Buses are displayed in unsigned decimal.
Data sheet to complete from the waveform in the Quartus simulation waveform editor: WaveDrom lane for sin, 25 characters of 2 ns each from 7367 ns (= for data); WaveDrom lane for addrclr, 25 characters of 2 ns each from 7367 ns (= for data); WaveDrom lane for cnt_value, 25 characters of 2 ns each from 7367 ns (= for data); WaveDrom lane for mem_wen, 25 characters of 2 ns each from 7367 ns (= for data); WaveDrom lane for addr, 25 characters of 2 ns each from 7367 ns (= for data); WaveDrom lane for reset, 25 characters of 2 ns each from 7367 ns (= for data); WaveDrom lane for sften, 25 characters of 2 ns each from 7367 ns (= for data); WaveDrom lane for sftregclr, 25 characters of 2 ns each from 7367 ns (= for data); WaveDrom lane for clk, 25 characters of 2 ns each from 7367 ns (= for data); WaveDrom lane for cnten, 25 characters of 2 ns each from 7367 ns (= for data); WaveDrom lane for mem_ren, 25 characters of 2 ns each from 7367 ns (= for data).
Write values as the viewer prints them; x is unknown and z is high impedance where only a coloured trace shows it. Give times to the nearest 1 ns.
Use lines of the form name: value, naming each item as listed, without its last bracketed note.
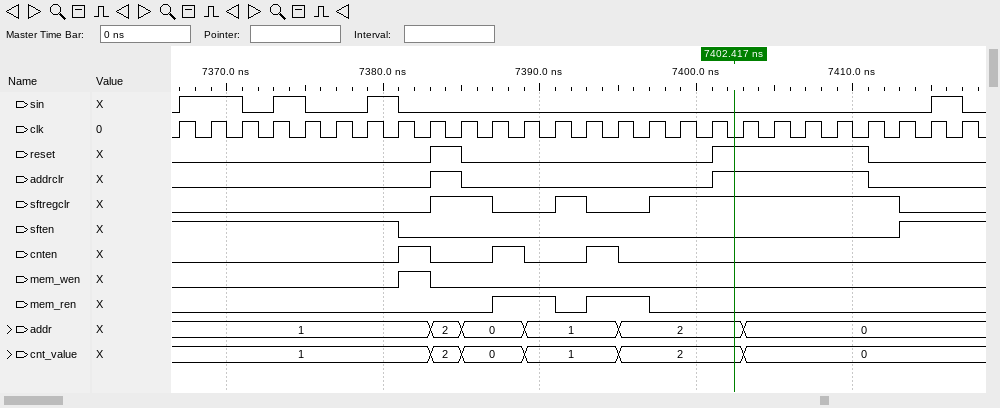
WaveDrom lane for sin, 25 characters of 2 ns each from 7367 ns: {name: 'sin', wave: '1.010.10................1'}
WaveDrom lane for addrclr, 25 characters of 2 ns each from 7367 ns: {name: 'addrclr', wave: '0.......10.......1....0..'}
WaveDrom lane for cnt_value, 25 characters of 2 ns each from 7367 ns: {name: 'cnt_value', wave: '=.......==.=..=...=......', data: '1 2 0 1 2 0'}
WaveDrom lane for mem_wen, 25 characters of 2 ns each from 7367 ns: {name: 'mem_wen', wave: '0......10................'}
WaveDrom lane for addr, 25 characters of 2 ns each from 7367 ns: {name: 'addr', wave: '=.......==.=..=...=......', data: '1 2 0 1 2 0'}
WaveDrom lane for reset, 25 characters of 2 ns each from 7367 ns: {name: 'reset', wave: '0.......10.......1....0..'}
WaveDrom lane for sften, 25 characters of 2 ns each from 7367 ns: {name: 'sften', wave: '1......0...............1.'}
WaveDrom lane for sftregclr, 25 characters of 2 ns each from 7367 ns: {name: 'sftregclr', wave: '0.......1.0.10.1.......0.'}
WaveDrom lane for clk, 25 characters of 2 ns each from 7367 ns: {name: 'clk', wave: 'p........................'}
WaveDrom lane for cnten, 25 characters of 2 ns each from 7367 ns: {name: 'cnten', wave: '0......10.10.10..........'}
WaveDrom lane for mem_ren, 25 characters of 2 ns each from 7367 ns: {name: 'mem_ren', wave: '0.........1.01.0.........'}
